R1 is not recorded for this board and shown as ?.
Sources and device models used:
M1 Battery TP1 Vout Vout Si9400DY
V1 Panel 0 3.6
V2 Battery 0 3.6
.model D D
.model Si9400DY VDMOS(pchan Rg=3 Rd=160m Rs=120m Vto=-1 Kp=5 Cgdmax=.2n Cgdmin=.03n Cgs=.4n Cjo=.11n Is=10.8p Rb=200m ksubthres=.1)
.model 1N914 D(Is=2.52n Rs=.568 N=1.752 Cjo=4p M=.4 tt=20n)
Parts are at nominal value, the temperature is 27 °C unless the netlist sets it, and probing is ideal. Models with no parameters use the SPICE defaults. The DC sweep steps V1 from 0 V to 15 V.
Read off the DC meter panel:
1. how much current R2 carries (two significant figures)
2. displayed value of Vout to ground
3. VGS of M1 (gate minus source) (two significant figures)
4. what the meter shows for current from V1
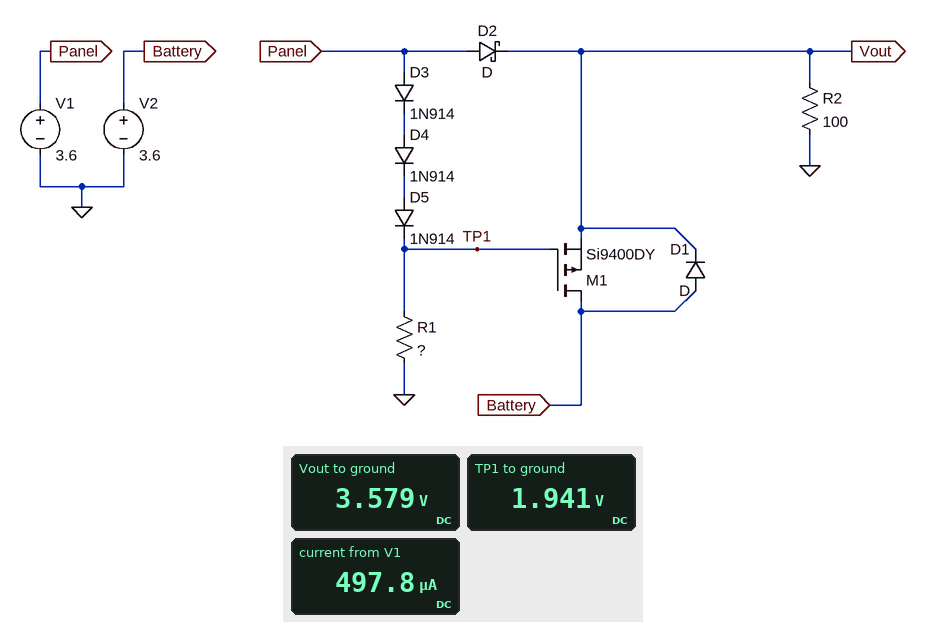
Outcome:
36 mA
3.579 V
-1.6 V
497.8 µA
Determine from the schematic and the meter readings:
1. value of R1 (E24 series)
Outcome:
3.9 kΩ
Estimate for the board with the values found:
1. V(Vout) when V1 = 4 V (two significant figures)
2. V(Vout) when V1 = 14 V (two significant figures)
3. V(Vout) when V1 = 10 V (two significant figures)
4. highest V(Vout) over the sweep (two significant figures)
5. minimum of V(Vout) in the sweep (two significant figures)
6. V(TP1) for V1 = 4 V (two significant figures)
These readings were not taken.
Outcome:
3.6 V
13 V
9.2 V
14 V
3.5 V
2.3 V
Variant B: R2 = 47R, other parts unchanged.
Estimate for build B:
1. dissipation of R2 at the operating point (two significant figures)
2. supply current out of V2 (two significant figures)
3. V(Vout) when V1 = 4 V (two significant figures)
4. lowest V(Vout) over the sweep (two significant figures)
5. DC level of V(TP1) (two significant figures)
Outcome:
270 mW
76 mA
3.5 V
3.4 V
1.9 V
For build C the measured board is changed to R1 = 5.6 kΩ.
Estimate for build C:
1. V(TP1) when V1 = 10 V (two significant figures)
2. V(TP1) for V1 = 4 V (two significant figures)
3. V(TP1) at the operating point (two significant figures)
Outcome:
8.2 V
2.4 V
2.0 V
